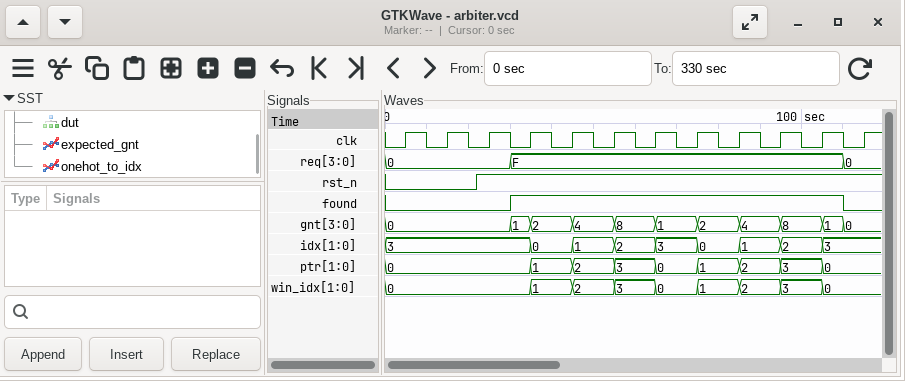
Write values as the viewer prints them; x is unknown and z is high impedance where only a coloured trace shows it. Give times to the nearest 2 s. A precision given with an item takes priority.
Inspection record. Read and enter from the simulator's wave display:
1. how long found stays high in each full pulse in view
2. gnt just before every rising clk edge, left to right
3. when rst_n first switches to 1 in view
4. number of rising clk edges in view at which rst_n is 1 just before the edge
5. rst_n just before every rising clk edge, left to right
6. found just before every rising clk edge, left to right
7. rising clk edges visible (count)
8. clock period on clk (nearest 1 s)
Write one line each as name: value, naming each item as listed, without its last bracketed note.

how long found stays high in each full pulse in view: 80 s
gnt just before every rising clk edge, left to right: 0, 0, 0, 1, 2, 4, 8, 1, 2, 4, 8, 0
when rst_n first switches to 1 in view: 22 s
number of rising clk edges in view at which rst_n is 1 just before the edge: 10
rst_n just before every rising clk edge, left to right: 0 0 1 1 1 1 1 1 1 1 1 1
found just before every rising clk edge, left to right: 0 0 0 1 1 1 1 1 1 1 1 0
rising clk edges visible: 12
clock period on clk: 10 s
